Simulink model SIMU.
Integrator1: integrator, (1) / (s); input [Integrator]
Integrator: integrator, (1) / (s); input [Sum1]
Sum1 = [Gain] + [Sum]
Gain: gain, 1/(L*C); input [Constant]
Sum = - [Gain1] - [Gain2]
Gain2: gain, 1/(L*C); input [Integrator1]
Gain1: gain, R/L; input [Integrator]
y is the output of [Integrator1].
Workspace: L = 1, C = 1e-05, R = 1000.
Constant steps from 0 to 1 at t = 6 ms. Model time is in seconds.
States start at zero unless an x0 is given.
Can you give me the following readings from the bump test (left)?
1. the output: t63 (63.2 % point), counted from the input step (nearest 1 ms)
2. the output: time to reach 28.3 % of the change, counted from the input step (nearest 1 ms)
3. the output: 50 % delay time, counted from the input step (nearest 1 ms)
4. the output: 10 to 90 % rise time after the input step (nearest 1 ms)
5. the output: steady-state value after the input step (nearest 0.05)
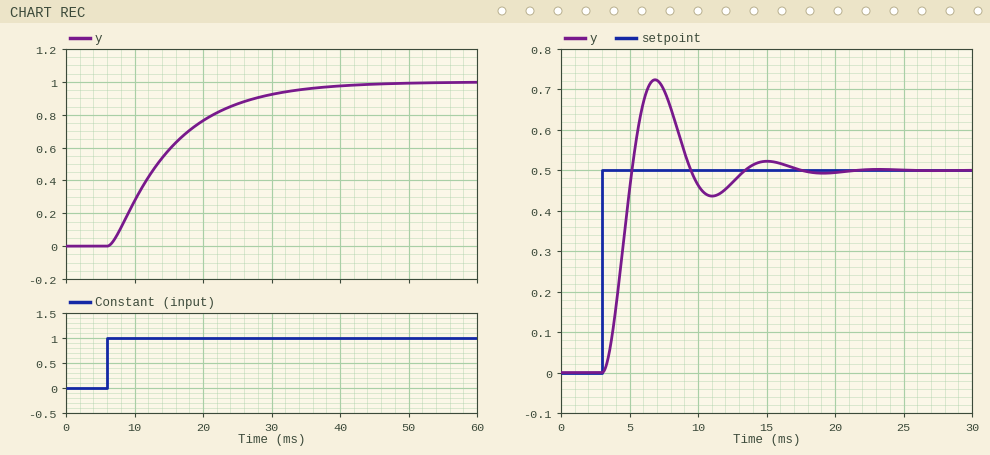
10 ms
4 ms
7 ms
20 ms
1.00
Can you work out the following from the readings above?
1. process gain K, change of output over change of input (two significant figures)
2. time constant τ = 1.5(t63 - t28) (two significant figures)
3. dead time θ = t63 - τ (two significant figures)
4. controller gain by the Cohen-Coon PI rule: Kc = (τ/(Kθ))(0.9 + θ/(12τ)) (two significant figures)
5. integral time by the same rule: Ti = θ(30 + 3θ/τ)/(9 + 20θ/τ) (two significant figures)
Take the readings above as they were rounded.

1.0
9.0 ms
1.0 ms
8.2
2.7 ms
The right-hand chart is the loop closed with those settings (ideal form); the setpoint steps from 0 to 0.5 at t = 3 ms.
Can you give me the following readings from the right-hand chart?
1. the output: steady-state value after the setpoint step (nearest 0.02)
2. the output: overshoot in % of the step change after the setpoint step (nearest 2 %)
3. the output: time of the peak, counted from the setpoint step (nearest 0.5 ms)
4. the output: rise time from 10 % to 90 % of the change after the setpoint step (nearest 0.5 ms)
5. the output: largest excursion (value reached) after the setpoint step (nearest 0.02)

0.50
44 %
4.0 ms
1.5 ms
0.72
